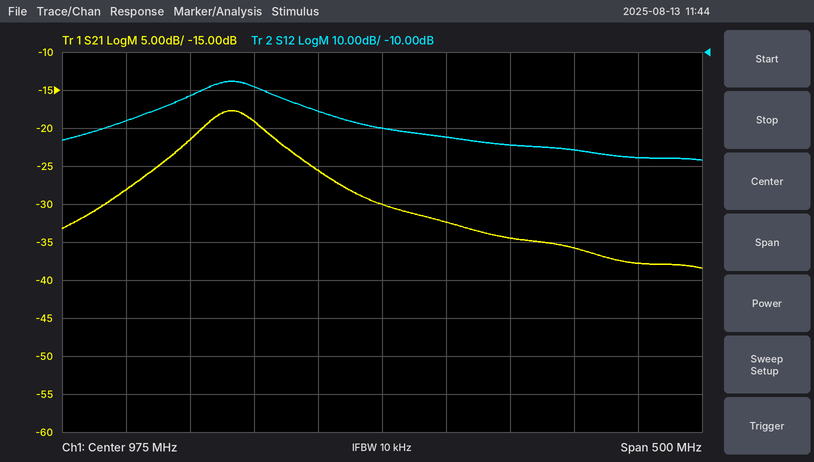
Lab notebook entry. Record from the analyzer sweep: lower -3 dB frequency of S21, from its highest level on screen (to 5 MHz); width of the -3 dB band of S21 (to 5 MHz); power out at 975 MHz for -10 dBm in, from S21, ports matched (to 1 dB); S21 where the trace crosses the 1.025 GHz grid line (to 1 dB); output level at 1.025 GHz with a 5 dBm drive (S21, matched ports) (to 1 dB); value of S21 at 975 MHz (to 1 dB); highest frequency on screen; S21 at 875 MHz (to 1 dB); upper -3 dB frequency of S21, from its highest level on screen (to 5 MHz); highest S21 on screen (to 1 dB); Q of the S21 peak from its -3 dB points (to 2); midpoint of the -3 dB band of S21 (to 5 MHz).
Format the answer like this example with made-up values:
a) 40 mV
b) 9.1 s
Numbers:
a) 830 MHz
b) 55 MHz
c) -40 dBm
d) -32 dB
e) -27 dBm
f) -30 dB
g) 1.225 GHz
h) -19 dB
i) 885 MHz
j) -18 dB
k) 16
l) 860 MHz
